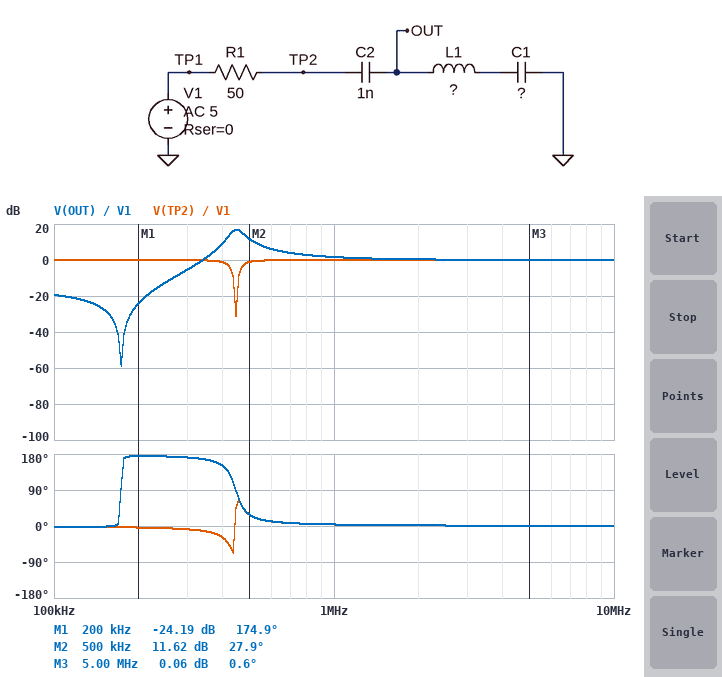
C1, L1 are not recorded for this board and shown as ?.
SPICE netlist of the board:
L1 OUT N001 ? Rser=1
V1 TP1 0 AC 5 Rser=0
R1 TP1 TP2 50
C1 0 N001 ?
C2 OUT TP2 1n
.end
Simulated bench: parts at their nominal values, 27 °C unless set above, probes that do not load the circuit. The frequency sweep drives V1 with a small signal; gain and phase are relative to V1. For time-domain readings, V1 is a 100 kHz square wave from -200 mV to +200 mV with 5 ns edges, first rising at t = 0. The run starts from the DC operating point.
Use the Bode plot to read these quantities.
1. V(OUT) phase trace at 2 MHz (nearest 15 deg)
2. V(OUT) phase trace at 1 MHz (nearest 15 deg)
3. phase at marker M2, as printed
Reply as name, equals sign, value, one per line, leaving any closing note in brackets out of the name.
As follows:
V(OUT) phase trace at 2 MHz = 0 deg
V(OUT) phase trace at 1 MHz = 0 deg
phase at marker M2, as printed = 27.9 deg
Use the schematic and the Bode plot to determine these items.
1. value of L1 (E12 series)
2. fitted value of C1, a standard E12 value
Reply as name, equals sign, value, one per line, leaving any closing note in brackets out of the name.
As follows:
value of L1 = 150 µH
fitted value of C1, a standard E12 value = 5.6 nF
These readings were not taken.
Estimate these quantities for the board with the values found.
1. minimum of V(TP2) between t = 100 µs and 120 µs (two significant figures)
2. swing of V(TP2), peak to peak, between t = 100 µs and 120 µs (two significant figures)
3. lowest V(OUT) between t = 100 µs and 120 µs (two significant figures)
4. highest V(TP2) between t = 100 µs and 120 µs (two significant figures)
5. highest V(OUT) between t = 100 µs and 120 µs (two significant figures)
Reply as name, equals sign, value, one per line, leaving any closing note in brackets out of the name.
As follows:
minimum of V(TP2) between t = 100 µs and 120 µs = -230 mV
swing of V(TP2), peak to peak, between t = 100 µs and 120 µs = 460 mV
lowest V(OUT) between t = 100 µs and 120 µs = -290 mV
highest V(TP2) between t = 100 µs and 120 µs = 230 mV
highest V(OUT) between t = 100 µs and 120 µs = 350 mV
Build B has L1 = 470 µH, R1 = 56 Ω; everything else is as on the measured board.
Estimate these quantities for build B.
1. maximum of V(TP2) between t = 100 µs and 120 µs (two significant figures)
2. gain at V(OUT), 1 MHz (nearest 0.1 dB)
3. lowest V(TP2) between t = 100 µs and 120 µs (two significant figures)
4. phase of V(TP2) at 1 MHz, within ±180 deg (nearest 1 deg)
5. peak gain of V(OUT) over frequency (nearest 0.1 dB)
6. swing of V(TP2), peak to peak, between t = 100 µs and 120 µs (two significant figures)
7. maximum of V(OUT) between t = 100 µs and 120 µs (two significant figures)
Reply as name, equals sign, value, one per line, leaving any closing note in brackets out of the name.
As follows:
maximum of V(TP2) between t = 100 µs and 120 µs = 220 mV
gain at V(OUT), 1 MHz = 0.5 dB
lowest V(TP2) between t = 100 µs and 120 µs = -220 mV
phase of V(TP2) at 1 MHz, within ±180 deg = 1 deg
peak gain of V(OUT) over frequency = 20.9 dB
swing of V(TP2), peak to peak, between t = 100 µs and 120 µs = 440 mV
maximum of V(OUT) between t = 100 µs and 120 µs = 340 mV
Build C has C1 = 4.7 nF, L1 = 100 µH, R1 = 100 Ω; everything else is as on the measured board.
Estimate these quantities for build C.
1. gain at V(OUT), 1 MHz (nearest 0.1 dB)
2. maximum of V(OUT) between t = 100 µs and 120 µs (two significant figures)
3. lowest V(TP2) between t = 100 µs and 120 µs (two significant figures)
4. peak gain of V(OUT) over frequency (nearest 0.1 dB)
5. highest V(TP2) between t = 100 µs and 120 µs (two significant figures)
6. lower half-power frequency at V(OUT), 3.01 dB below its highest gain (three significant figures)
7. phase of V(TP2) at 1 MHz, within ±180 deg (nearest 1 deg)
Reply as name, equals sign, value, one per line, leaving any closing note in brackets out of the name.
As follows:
gain at V(OUT), 1 MHz = 2.5 dB
maximum of V(OUT) between t = 100 µs and 120 µs = 390 mV
lowest V(TP2) between t = 100 µs and 120 µs = -260 mV
peak gain of V(OUT) over frequency = 9.3 dB
highest V(TP2) between t = 100 µs and 120 µs = 260 mV
lower half-power frequency at V(OUT), 3.01 dB below its highest gain = 503 kHz
phase of V(TP2) at 1 MHz, within ±180 deg = 13 deg
